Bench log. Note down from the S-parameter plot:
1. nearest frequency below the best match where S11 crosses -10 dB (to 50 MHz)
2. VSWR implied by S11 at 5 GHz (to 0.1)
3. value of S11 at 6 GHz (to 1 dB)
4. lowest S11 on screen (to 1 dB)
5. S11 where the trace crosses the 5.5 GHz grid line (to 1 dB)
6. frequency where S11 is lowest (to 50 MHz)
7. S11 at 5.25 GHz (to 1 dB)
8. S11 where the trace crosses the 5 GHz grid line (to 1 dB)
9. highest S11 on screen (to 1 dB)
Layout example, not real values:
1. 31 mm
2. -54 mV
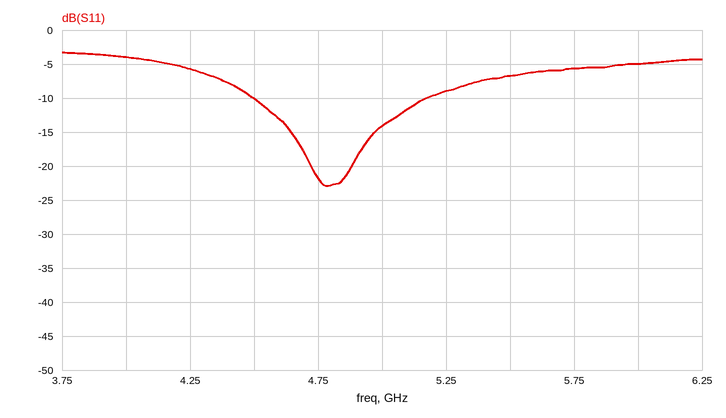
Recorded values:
1. 4.50 GHz
2. 1.5
3. -5 dB
4. -23 dB
5. -7 dB
6. 4.80 GHz
7. -9 dB
8. -14 dB
9. -3 dB
